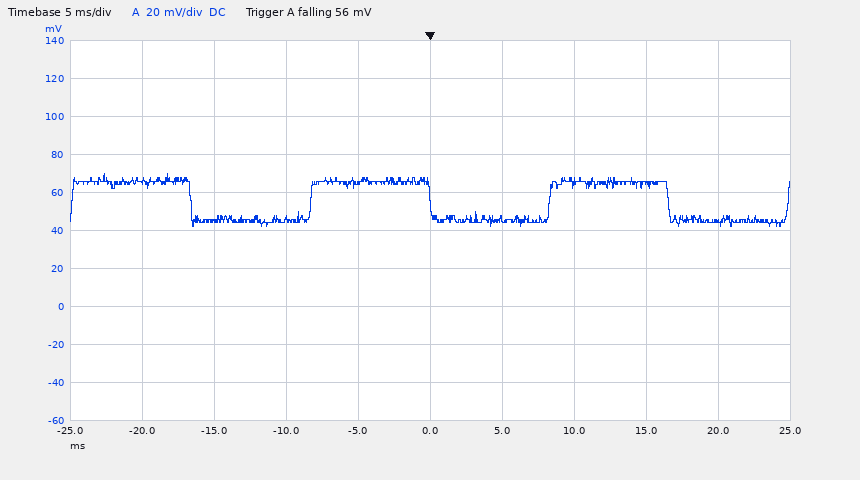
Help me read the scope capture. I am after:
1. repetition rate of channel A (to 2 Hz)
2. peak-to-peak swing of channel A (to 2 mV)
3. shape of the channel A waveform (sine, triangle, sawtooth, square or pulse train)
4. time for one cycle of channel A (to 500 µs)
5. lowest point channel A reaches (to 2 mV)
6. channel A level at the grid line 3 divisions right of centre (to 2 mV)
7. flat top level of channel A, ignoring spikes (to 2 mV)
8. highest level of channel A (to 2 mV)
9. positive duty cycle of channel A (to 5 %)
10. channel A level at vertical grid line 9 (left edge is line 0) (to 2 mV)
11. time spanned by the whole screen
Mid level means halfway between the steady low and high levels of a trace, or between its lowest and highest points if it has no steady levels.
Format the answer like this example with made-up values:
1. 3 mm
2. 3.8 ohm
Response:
1. 60 Hz
2. 28 mV
3. square
4. 16.5 ms
5. 42 mV
6. 64 mV
7. 66 mV
8. 70 mV
9. 50 %
10. 44 mV
11. 50 ms
